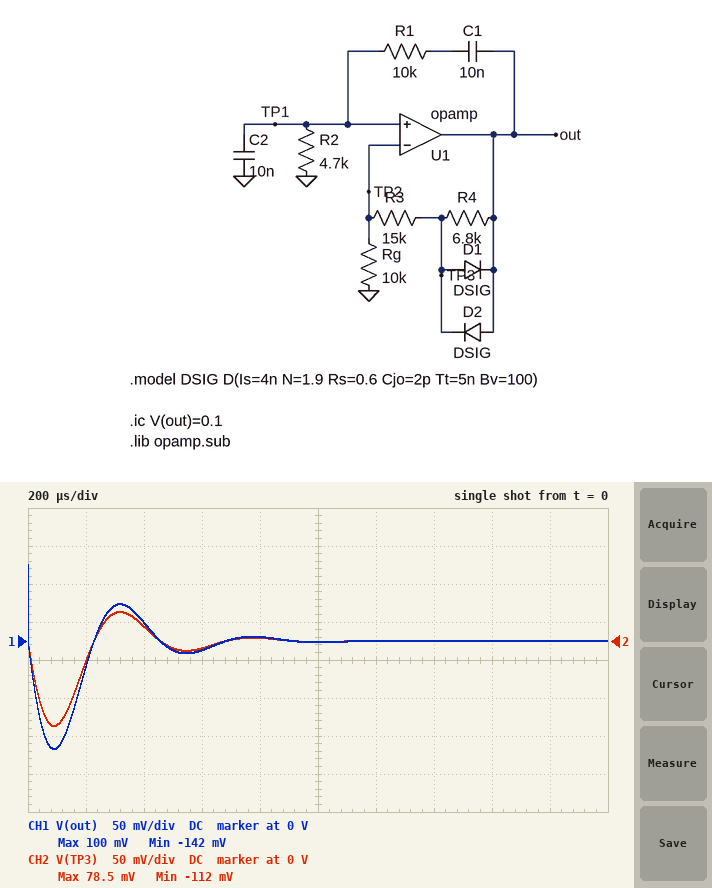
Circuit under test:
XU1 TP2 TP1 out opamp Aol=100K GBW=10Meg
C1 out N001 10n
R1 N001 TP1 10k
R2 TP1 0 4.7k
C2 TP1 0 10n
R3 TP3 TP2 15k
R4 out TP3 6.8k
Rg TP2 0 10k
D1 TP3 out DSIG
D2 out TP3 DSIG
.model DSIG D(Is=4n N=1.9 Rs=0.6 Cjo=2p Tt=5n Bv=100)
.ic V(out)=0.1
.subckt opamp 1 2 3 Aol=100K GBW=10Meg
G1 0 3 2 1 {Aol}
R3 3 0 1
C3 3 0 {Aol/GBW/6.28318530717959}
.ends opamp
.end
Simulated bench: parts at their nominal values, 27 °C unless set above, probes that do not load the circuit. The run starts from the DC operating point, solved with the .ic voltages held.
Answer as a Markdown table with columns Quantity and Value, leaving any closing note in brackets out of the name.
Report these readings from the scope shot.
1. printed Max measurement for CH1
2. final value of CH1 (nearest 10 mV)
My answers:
| Quantity | Value |
|---|---|
| printed Max measurement for CH1 | 100 mV |
| final value of CH1 | 0 V |
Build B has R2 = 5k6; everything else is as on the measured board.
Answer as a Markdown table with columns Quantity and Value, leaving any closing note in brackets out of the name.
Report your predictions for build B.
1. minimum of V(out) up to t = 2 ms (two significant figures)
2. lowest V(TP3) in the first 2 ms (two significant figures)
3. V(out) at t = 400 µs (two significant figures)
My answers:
| Quantity | Value |
|---|---|
| minimum of V(out) up to t = 2 ms | -170 mV |
| lowest V(TP3) in the first 2 ms | -140 mV |
| V(out) at t = 400 µs | 64 mV |
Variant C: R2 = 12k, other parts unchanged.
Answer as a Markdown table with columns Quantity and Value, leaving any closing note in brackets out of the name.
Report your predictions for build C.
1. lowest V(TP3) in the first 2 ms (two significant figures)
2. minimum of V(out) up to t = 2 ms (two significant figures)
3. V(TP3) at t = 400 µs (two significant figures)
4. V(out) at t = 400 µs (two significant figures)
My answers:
| Quantity | Value |
|---|---|
| lowest V(TP3) in the first 2 ms | -2.7 V |
| minimum of V(out) up to t = 2 ms | -3.2 V |
| V(TP3) at t = 400 µs | 240 mV |
| V(out) at t = 400 µs | 300 mV |
